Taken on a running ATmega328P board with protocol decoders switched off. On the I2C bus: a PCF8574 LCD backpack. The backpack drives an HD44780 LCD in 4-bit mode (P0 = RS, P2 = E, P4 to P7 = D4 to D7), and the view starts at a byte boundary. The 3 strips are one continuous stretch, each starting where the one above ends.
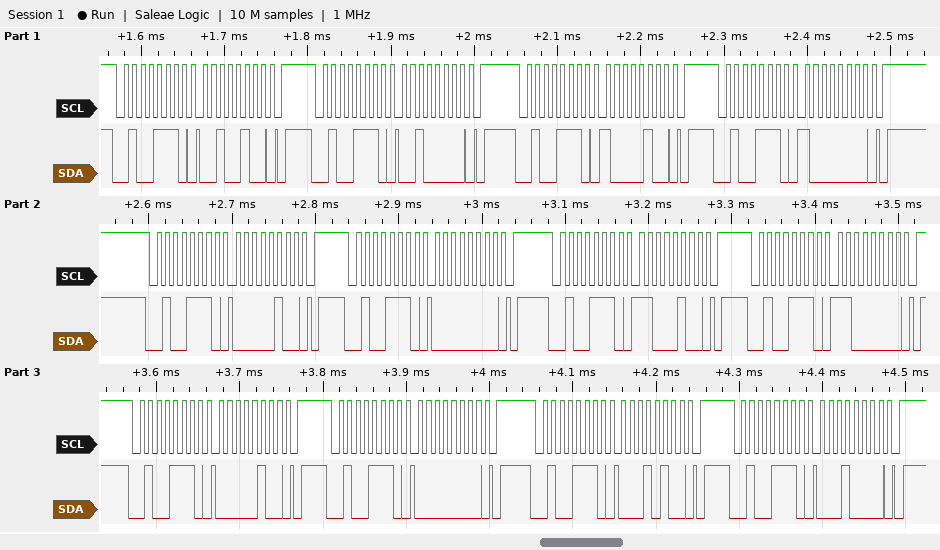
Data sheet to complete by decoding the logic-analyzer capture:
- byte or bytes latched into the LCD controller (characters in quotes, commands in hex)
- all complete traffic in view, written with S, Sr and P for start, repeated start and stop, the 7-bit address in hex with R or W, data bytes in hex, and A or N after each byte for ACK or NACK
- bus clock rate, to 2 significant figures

0x28 0x0C 0x01
S 27W A 24 A P S 27W A 20 A P S 27W A 84 A P S 27W A 80 A P S 27W A 04 A P S 27W A 00 A P S 27W A C4 A P S 27W A C0 A P S 27W A 04 A P S 27W A 00 A P S 27W A 14 A P S 27W A 10 A P
100 kHz
